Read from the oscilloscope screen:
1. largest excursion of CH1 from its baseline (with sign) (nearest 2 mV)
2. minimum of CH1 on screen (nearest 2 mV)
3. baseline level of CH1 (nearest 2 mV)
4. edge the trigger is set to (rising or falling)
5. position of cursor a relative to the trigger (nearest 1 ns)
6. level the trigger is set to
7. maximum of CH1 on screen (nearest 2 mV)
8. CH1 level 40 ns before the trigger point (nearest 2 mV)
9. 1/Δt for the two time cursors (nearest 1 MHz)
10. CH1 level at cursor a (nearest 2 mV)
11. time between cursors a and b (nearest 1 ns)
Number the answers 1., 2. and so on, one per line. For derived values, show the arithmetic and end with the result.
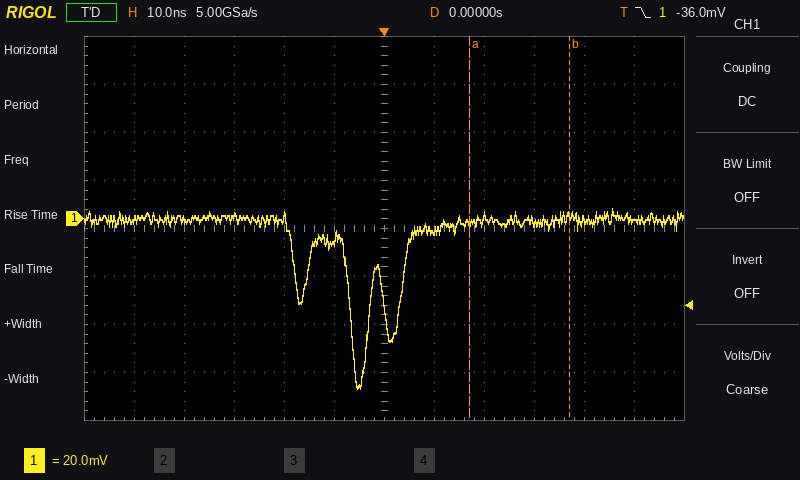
1. -70 mV − (0 mV) = -70 mV
2. -70 mV
3. 0 mV
4. falling
5. +17 ns
6. -36.0 mV
7. 4 mV
8. 0 mV
9. 1 / 20 ns ≈ 50 MHz
10. -2 mV
11. 20 ns
